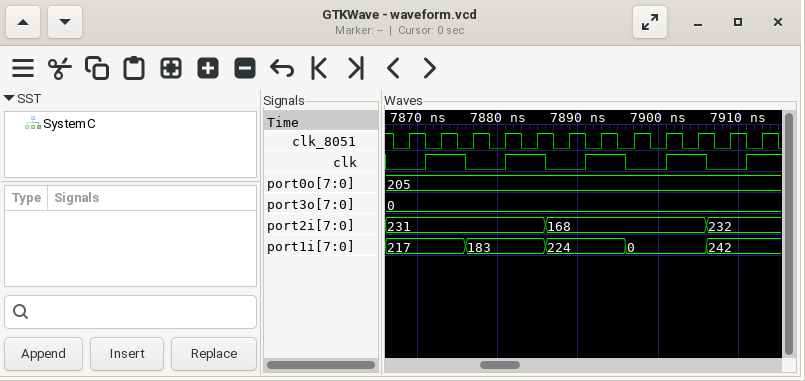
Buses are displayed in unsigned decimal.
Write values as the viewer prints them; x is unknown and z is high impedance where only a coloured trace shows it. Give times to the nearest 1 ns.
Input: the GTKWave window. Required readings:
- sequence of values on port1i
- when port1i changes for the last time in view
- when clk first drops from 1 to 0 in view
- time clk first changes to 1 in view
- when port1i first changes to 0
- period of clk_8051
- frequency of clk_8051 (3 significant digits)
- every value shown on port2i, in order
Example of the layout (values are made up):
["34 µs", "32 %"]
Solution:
["217, 183, 224, 0, 242", "7906 ns", "7876 ns", "7871 ns", "7896 ns", "4 ns", "250 MHz", "231, 168, 232"]
